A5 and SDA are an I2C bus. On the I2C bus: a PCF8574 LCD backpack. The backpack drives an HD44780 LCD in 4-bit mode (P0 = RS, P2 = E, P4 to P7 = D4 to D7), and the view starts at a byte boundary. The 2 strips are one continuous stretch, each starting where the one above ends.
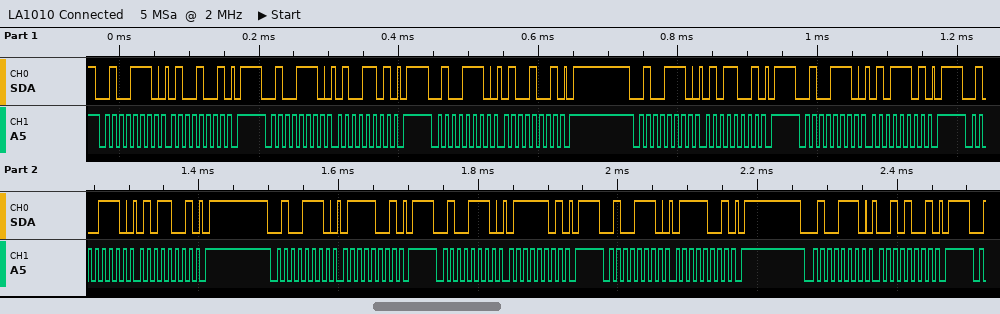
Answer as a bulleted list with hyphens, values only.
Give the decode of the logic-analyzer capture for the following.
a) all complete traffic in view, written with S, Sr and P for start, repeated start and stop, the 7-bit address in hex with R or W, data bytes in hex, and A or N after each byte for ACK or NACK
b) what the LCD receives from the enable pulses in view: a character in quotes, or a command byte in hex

- S 27W A 49 A P S 27W A 4D A P S 27W A 49 A P S 27W A 59 A P S 27W A 5D A P S 27W A 59 A P S 27W A 79 A P S 27W A 7D A P S 27W A 79 A P S 27W A 29 A P
- 'E'
